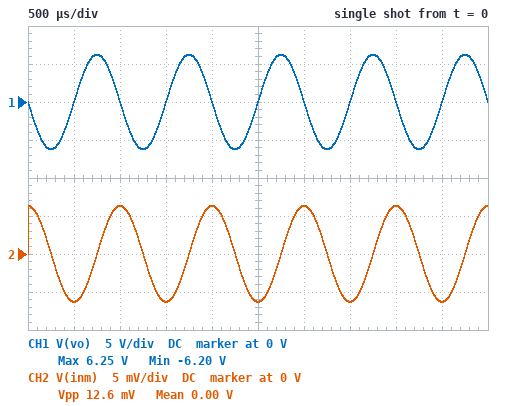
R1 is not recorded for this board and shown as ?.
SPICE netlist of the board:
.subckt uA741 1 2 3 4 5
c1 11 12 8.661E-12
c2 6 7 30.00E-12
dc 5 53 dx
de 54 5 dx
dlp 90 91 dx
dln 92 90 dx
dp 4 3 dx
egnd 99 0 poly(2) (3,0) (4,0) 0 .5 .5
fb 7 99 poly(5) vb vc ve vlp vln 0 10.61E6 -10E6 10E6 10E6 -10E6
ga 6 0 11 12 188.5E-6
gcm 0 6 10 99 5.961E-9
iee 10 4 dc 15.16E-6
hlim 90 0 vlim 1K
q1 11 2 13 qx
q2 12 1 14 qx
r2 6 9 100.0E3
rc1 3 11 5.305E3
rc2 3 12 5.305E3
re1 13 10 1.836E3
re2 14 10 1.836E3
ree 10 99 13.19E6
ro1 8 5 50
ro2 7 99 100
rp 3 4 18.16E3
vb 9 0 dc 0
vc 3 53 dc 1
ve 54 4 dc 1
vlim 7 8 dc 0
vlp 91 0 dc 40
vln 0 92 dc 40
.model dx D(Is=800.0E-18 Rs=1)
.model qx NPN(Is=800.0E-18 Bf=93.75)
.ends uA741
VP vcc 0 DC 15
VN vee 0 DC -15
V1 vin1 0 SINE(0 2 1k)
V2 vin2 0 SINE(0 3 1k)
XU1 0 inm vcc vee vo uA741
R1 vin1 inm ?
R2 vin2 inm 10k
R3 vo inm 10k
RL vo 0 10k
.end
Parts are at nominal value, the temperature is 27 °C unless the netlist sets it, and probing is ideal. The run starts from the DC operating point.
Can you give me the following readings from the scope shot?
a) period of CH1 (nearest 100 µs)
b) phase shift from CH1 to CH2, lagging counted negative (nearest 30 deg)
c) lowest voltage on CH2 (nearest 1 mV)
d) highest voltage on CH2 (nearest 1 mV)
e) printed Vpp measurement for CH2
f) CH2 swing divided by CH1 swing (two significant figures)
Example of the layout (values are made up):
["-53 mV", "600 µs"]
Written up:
["1.0 ms", "-90 deg", "-6 mV", "6 mV", "12.6 mV", "0.0010"]
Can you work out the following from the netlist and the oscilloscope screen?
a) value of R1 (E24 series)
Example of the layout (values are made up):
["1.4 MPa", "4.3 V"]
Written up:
["6.2 kΩ"]
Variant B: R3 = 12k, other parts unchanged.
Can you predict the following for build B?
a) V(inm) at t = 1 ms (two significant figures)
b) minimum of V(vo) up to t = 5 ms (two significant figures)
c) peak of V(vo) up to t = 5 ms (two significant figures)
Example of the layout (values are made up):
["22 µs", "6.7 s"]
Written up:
["7.6 mV", "-7.5 V", "7.5 V"]
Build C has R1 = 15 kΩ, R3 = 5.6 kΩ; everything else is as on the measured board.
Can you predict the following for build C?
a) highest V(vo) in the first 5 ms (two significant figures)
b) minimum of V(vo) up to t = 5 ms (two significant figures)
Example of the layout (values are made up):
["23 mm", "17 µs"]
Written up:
["2.4 V", "-2.4 V"]
